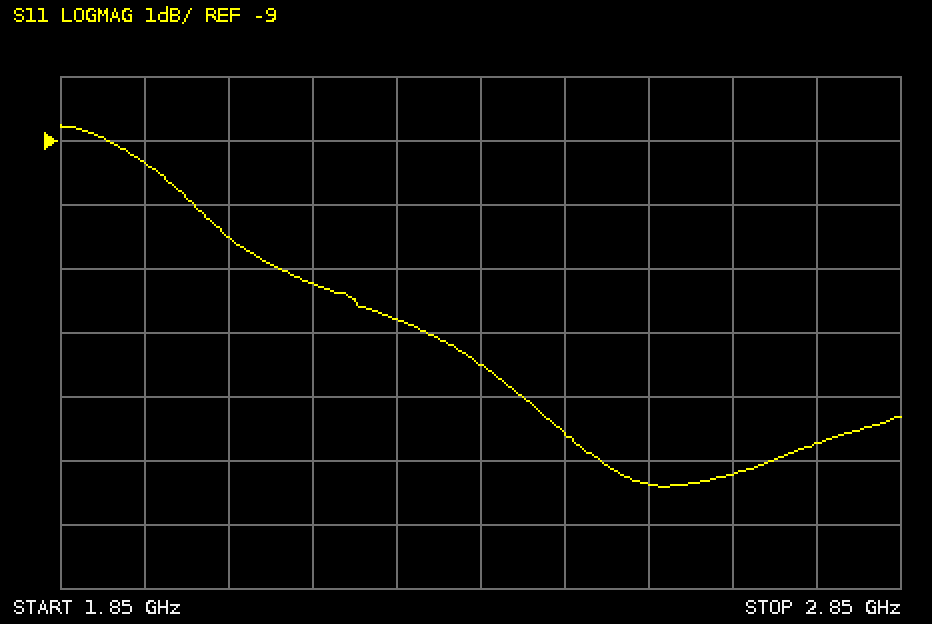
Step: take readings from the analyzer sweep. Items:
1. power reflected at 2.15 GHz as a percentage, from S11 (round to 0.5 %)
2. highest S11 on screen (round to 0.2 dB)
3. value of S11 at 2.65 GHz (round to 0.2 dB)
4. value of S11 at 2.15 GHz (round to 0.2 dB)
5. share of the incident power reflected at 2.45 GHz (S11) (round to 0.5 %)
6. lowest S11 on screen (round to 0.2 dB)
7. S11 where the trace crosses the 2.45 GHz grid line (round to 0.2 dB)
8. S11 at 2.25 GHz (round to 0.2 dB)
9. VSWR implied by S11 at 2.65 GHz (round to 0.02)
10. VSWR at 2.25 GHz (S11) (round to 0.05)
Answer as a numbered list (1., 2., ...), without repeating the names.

1. 7.5 %
2. -8.8 dB
3. -14.2 dB
4. -11.2 dB
5. 4.5 %
6. -14.4 dB
7. -13.6 dB
8. -11.8 dB
9. 1.48
10. 1.70
